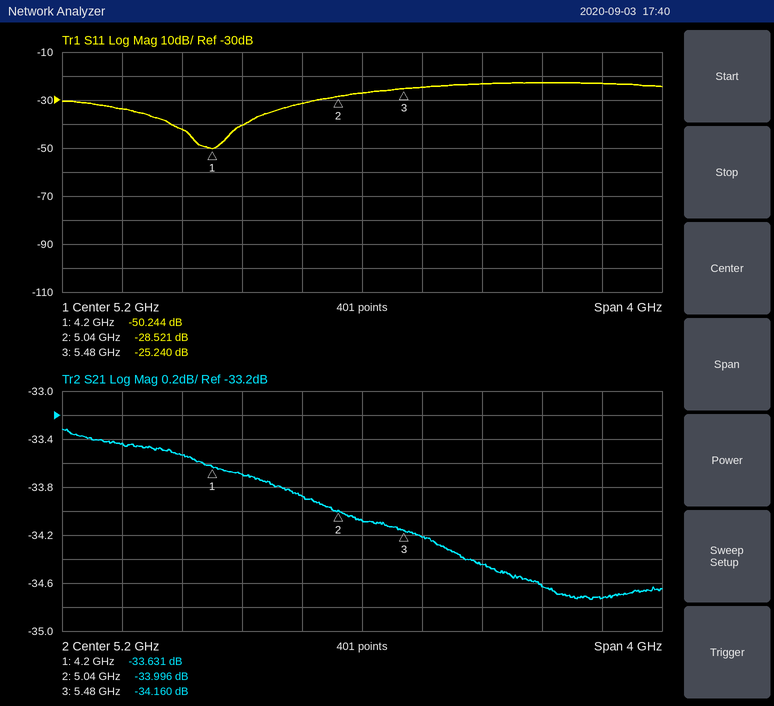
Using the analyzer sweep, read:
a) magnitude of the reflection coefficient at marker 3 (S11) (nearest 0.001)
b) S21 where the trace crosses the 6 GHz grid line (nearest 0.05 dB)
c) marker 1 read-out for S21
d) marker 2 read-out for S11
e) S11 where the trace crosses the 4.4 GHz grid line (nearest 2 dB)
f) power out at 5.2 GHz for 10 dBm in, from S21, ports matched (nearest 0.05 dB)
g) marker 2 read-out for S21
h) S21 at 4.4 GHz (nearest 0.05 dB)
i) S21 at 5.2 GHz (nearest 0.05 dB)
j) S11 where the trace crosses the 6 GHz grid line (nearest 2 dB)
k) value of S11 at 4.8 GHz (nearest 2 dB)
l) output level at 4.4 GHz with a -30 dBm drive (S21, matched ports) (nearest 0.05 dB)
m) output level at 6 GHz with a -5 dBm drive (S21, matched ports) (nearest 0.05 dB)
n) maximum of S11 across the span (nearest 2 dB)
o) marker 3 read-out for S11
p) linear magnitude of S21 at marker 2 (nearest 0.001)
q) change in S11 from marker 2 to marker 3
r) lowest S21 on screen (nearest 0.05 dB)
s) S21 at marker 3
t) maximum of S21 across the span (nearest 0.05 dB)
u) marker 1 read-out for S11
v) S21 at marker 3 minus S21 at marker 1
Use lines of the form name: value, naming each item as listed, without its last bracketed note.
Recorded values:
magnitude of the reflection coefficient at marker 3 (S11): 0.055
S21 where the trace crosses the 6 GHz grid line: -34.45 dB
marker 1 read-out for S21: -33.631 dB
marker 2 read-out for S11: -28.521 dB
S11 where the trace crosses the 4.4 GHz grid line: -40 dB
power out at 5.2 GHz for 10 dBm in, from S21, ports matched: -24.10 dBm
marker 2 read-out for S21: -33.996 dB
S21 at 4.4 GHz: -33.70 dB
S21 at 5.2 GHz: -34.10 dB
S11 where the trace crosses the 6 GHz grid line: -24 dB
value of S11 at 4.8 GHz: -32 dB
output level at 4.4 GHz with a -30 dBm drive (S21, matched ports): -63.70 dBm
output level at 6 GHz with a -5 dBm drive (S21, matched ports): -39.45 dBm
maximum of S11 across the span: -22 dB
marker 3 read-out for S11: -25.240 dB
linear magnitude of S21 at marker 2: 0.020
change in S11 from marker 2 to marker 3: 3.281 dB
lowest S21 on screen: -34.75 dB
S21 at marker 3: -34.160 dB
maximum of S21 across the span: -33.30 dB
marker 1 read-out for S11: -50.244 dB
S21 at marker 3 minus S21 at marker 1: -0.529 dB
